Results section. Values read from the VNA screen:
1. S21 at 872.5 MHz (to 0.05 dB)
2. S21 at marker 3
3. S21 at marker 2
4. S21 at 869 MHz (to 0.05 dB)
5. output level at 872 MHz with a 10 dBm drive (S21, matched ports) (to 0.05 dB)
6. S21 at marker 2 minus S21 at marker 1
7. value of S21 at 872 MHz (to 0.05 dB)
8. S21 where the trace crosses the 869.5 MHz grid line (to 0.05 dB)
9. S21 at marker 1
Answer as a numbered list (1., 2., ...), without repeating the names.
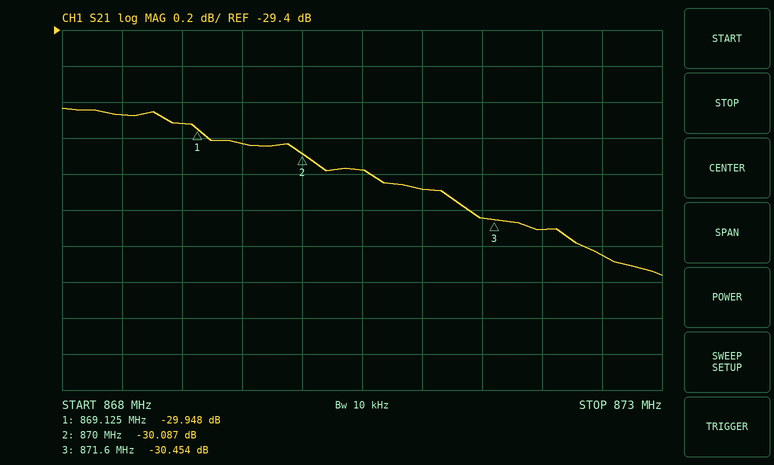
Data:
1. -30.65 dB
2. -30.454 dB
3. -30.087 dB
4. -29.90 dB
5. -20.50 dBm
6. -0.139 dB
7. -30.50 dB
8. -30.05 dB
9. -29.948 dB
